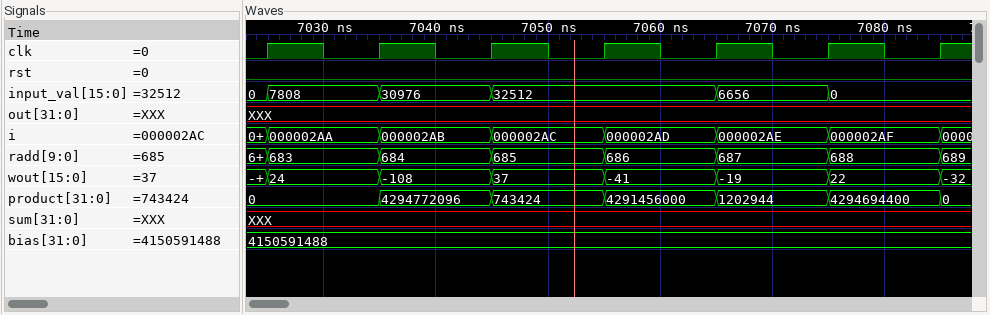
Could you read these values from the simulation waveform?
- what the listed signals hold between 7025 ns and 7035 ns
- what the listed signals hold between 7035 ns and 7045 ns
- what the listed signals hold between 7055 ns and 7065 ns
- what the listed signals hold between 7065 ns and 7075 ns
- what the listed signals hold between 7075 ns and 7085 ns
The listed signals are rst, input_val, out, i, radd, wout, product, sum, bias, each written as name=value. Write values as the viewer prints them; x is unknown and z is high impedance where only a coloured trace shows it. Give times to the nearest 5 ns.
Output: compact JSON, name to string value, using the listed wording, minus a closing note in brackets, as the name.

{"what the listed signals hold between 7025 ns and 7035 ns": "rst=0, input_val=7808, out=XXX, i=000002AA, radd=683, wout=24, product=0, sum=XXX, bias=4150591488", "what the listed signals hold between 7035 ns and 7045 ns": "rst=0, input_val=30976, out=XXX, i=000002AB, radd=684, wout=-108, product=4294772096, sum=XXX, bias=4150591488", "what the listed signals hold between 7055 ns and 7065 ns": "rst=0, input_val=32512, out=XXX, i=000002AD, radd=686, wout=-41, product=4291456000, sum=XXX, bias=4150591488", "what the listed signals hold between 7065 ns and 7075 ns": "rst=0, input_val=6656, out=XXX, i=000002AE, radd=687, wout=-19, product=1202944, sum=XXX, bias=4150591488", "what the listed signals hold between 7075 ns and 7085 ns": "rst=0, input_val=0, out=XXX, i=000002AF, radd=688, wout=22, product=4294694400, sum=XXX, bias=4150591488"}
